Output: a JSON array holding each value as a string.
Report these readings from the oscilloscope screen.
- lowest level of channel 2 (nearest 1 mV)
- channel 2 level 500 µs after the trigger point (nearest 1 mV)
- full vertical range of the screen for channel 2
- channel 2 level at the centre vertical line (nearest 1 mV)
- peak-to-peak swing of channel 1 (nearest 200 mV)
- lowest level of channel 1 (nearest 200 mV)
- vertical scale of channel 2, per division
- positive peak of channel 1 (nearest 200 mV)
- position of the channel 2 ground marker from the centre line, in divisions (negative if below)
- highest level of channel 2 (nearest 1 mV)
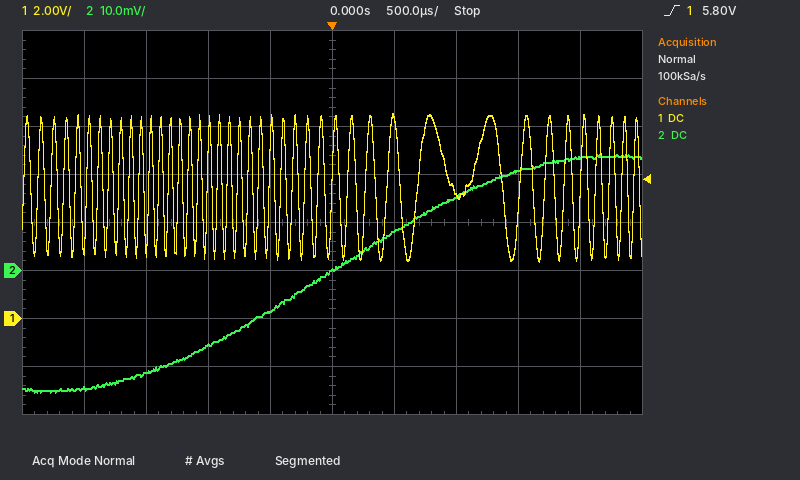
["-25 mV", "8 mV", "80 mV", "0 mV", "6.2 V", "2.4 V", "10 mV", "8.6 V", "-1.0 div", "24 mV"]
